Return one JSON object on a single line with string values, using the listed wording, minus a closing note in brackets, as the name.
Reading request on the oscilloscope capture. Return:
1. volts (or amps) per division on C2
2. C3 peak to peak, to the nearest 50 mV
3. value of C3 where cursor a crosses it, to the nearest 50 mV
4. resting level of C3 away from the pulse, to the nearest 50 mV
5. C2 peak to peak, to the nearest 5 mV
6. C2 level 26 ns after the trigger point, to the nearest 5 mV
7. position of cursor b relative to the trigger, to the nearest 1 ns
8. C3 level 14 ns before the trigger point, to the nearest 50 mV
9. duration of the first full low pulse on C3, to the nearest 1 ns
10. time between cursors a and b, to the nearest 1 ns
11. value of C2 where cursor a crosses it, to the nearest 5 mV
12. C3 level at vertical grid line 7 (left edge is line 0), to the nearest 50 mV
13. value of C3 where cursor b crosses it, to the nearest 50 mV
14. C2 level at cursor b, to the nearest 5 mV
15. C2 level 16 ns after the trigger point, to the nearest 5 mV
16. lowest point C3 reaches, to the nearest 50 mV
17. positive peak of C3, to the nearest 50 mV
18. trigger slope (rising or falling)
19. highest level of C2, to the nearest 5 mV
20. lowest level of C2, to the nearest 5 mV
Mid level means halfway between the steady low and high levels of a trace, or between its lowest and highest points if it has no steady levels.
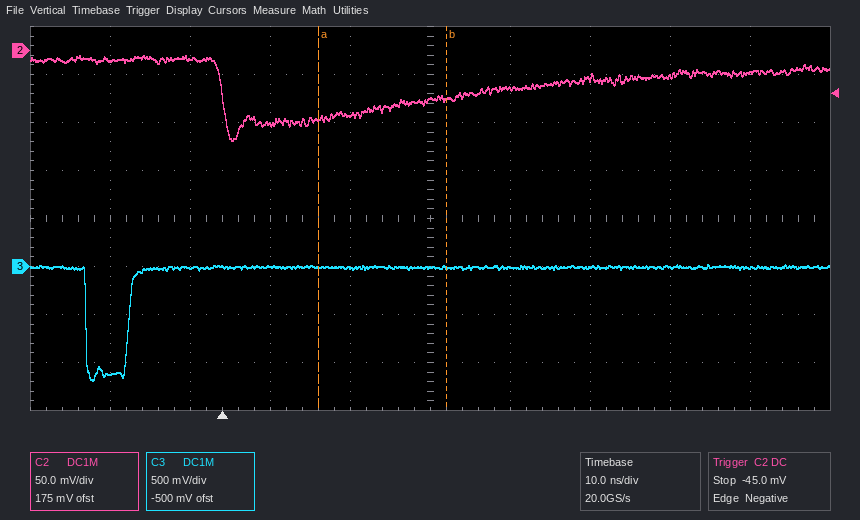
{"volts (or amps) per division on C2": "50 mV", "C3 peak to peak, to the nearest 50 mV": "1.20 V", "value of C3 where cursor a crosses it, to the nearest 50 mV": "0 mV", "resting level of C3 away from the pulse, to the nearest 50 mV": "0 mV", "C2 peak to peak, to the nearest 5 mV": "90 mV", "C2 level 26 ns after the trigger point, to the nearest 5 mV": "-50 mV", "position of cursor b relative to the trigger, to the nearest 1 ns": "+28 ns", "C3 level 14 ns before the trigger point, to the nearest 50 mV": "-1.10 V", "duration of the first full low pulse on C3, to the nearest 1 ns": "5 ns", "time between cursors a and b, to the nearest 1 ns": "16 ns", "value of C2 where cursor a crosses it, to the nearest 5 mV": "-70 mV", "C3 level at vertical grid line 7 (left edge is line 0), to the nearest 50 mV": "0 mV", "value of C3 where cursor b crosses it, to the nearest 50 mV": "0 mV", "C2 level at cursor b, to the nearest 5 mV": "-50 mV", "C2 level 16 ns after the trigger point, to the nearest 5 mV": "-65 mV", "lowest point C3 reaches, to the nearest 50 mV": "-1.20 V", "positive peak of C3, to the nearest 50 mV": "0 mV", "trigger slope": "falling", "highest level of C2, to the nearest 5 mV": "-5 mV", "lowest level of C2, to the nearest 5 mV": "-95 mV"}
